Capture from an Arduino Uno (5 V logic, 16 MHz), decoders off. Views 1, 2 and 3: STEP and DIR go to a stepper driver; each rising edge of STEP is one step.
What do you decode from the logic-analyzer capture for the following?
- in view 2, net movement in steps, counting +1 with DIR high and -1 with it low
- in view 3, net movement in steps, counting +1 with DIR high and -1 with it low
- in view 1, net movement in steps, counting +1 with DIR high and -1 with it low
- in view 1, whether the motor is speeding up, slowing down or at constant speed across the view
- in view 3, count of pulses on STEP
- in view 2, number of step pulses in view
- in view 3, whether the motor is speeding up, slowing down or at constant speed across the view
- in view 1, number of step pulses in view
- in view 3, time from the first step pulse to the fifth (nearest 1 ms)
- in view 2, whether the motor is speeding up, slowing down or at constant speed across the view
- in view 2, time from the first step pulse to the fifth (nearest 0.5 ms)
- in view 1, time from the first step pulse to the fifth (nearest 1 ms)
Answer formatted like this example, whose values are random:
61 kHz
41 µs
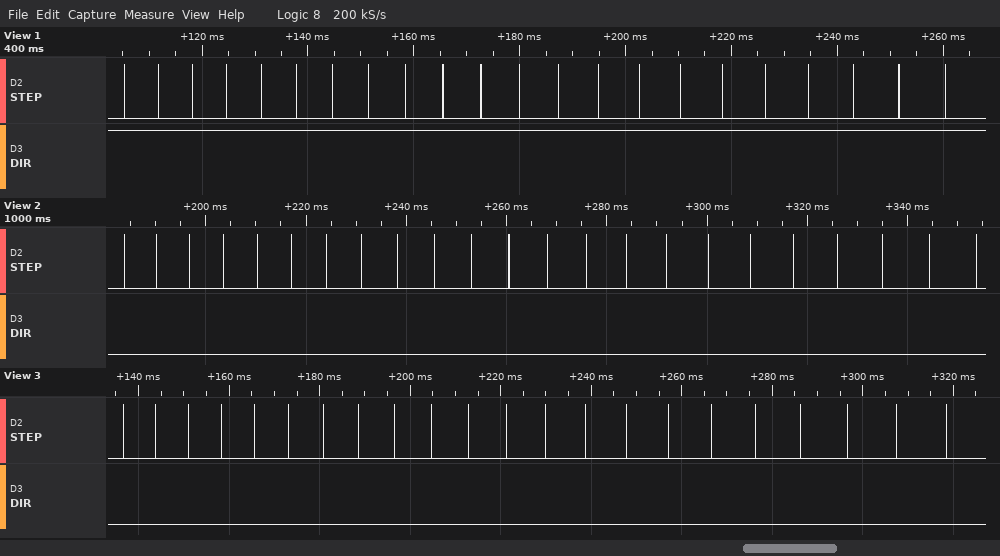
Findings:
-23
-22
+22
slowing down
22
23
slowing down
22
29 ms
slowing down
26.5 ms
26 ms
